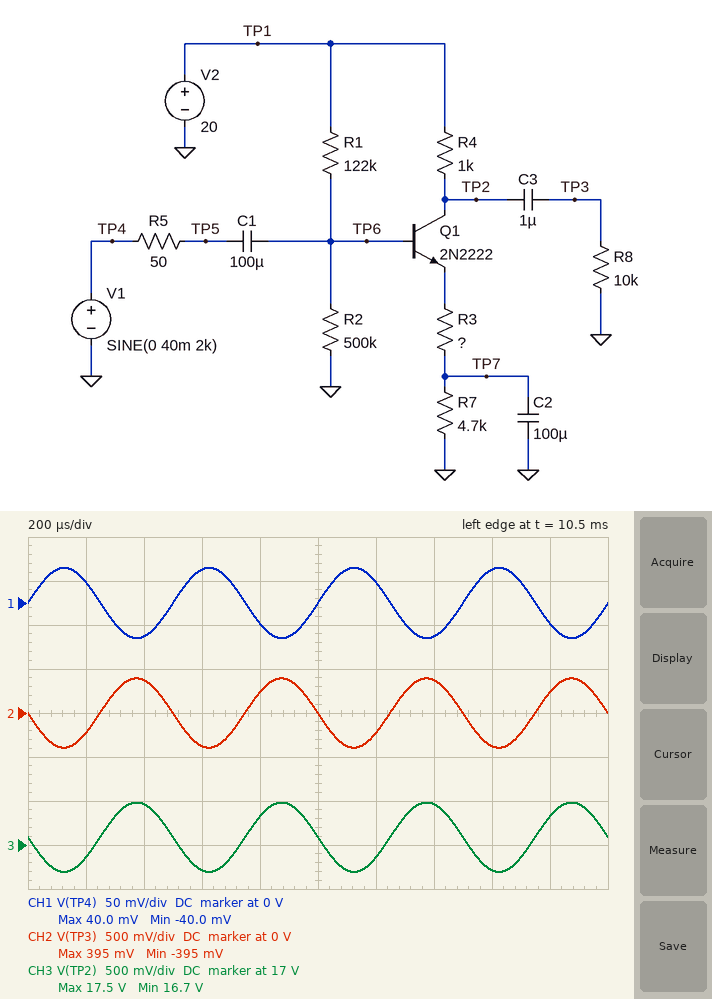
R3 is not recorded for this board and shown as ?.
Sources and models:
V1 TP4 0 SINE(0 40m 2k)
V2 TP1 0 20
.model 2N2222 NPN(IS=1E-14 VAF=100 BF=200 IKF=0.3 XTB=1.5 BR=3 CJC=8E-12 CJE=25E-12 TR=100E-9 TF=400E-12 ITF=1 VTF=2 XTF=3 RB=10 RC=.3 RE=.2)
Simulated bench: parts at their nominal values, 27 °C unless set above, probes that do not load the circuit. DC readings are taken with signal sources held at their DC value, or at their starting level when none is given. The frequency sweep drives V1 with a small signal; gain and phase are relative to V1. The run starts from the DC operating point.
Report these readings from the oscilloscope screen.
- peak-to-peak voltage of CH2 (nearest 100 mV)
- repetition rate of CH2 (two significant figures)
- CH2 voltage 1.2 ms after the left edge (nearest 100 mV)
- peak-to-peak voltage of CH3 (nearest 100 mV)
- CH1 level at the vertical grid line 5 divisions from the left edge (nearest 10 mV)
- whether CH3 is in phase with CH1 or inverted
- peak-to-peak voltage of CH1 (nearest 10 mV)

800 mV
2.0 kHz
-200 mV
800 mV
0 V
inverted
80 mV
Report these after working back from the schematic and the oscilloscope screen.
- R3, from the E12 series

82 Ω
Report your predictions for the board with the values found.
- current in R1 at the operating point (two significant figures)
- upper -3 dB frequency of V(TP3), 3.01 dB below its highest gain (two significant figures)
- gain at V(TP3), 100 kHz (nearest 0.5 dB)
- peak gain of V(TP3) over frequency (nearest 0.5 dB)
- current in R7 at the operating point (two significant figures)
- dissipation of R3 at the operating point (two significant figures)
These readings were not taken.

44 µA
19 MHz
20.0 dB
20.0 dB
2.9 mA
700 µW
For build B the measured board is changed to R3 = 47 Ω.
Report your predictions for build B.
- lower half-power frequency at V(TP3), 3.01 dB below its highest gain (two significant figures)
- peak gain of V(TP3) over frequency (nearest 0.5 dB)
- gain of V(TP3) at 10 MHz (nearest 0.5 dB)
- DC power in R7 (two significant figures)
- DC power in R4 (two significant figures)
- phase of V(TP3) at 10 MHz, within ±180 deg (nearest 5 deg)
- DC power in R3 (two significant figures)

34 Hz
24.0 dB
22.5 dB
41 mW
8.6 mW
145 deg
410 µW
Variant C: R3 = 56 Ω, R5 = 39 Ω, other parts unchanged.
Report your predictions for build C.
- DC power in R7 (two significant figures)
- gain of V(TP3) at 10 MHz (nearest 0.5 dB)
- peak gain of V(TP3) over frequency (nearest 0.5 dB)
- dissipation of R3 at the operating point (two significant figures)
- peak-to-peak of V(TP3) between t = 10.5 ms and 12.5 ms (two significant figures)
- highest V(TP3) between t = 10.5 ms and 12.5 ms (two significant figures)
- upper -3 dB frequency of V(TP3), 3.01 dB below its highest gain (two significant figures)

41 mW
21.5 dB
23.0 dB
480 µW
1.1 V
550 mV
18 MHz
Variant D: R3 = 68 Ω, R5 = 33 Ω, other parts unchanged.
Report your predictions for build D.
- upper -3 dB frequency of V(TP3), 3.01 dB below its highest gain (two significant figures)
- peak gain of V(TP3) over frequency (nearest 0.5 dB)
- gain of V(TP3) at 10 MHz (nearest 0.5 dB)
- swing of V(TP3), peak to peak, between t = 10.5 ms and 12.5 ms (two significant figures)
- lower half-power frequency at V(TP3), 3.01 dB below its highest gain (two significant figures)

21 MHz
21.5 dB
20.5 dB
930 mV
28 Hz
